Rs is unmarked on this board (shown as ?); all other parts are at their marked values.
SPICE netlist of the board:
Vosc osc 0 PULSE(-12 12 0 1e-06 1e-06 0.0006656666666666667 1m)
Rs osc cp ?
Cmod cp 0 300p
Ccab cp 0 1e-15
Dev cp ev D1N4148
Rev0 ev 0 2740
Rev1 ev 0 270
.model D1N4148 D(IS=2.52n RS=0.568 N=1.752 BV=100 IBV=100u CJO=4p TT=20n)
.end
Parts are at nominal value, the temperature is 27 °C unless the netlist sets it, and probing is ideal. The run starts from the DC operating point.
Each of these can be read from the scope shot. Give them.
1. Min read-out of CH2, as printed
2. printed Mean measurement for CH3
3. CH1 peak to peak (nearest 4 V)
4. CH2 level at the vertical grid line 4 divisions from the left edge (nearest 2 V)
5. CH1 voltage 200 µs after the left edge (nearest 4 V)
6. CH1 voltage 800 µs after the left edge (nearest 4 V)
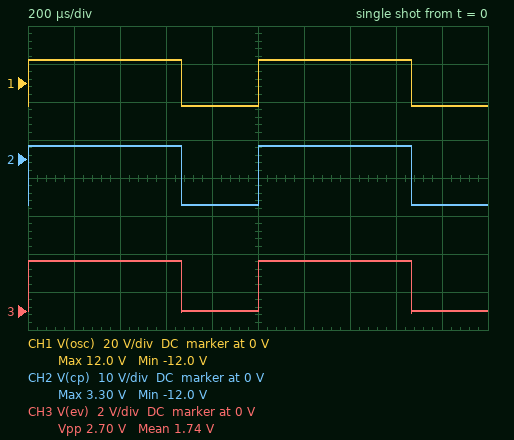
-12.0 V
1.74 V
24 V
-12 V
12 V
-12 V
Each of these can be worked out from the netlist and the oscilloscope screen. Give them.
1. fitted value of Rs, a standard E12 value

820 Ω
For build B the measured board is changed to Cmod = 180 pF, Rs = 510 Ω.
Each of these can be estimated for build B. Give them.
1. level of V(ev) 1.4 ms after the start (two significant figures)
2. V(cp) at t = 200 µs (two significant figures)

3.7 V
4.4 V
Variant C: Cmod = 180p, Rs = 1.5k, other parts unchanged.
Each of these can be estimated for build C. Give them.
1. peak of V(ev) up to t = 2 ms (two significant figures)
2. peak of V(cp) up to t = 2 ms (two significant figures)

1.6 V
2.3 V
